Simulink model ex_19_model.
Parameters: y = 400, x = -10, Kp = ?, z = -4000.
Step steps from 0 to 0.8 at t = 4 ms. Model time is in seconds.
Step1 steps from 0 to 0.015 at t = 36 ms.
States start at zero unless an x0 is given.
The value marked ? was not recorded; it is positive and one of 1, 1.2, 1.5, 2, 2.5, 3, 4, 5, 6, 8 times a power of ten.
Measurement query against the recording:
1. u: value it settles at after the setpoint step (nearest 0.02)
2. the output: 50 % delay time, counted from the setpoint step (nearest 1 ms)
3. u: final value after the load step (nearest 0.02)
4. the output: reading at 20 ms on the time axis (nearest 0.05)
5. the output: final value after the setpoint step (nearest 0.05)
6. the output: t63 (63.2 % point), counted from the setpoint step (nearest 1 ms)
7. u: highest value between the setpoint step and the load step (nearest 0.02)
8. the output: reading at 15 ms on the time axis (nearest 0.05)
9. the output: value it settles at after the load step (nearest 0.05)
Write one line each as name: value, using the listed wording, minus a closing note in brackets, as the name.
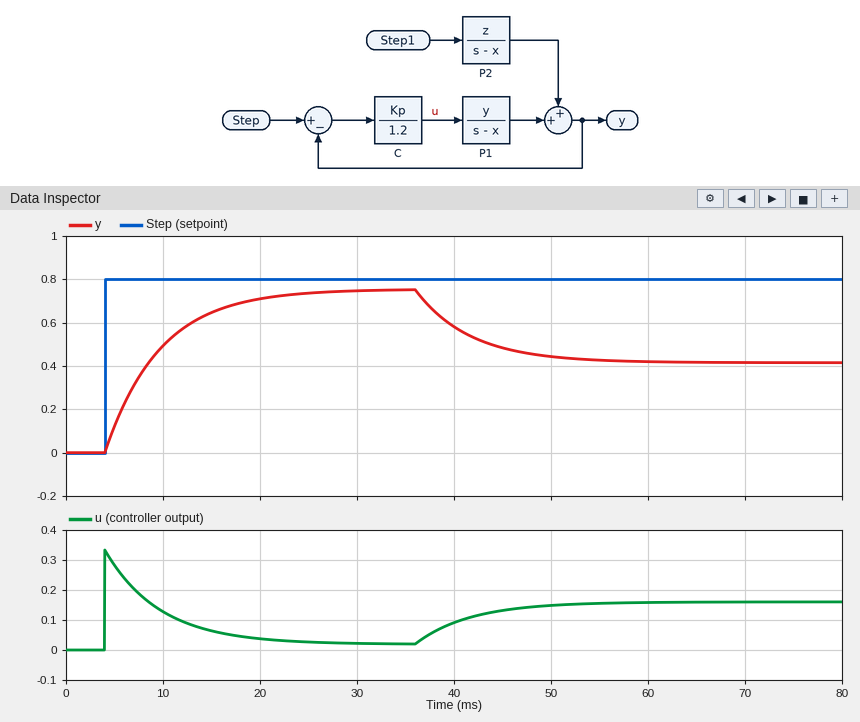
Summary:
u: value it settles at after the setpoint step: 0.02
the output: 50 % delay time, counted from the setpoint step: 4 ms
u: final value after the load step: 0.16
the output: reading at 20 ms on the time axis: 0.70
the output: final value after the setpoint step: 0.75
the output: t63 (63.2 % point), counted from the setpoint step: 6 ms
u: highest value between the setpoint step and the load step: 0.34
the output: reading at 15 ms on the time axis: 0.65
the output: value it settles at after the load step: 0.40
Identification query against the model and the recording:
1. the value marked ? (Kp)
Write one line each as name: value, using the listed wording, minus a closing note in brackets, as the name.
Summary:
the value marked ?: 0.5
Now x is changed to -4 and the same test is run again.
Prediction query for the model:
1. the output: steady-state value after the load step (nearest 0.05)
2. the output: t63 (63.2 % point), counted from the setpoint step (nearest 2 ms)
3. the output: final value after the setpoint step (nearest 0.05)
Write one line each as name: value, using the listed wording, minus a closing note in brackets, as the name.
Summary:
the output: steady-state value after the load step: 0.45
the output: t63 (63.2 % point), counted from the setpoint step: 6 ms
the output: final value after the setpoint step: 0.80
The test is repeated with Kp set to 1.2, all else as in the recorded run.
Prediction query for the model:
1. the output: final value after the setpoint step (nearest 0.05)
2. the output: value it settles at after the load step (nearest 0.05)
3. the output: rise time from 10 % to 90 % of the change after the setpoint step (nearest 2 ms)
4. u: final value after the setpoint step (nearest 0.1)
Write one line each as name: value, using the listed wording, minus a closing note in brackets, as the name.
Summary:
the output: final value after the setpoint step: 0.80
the output: value it settles at after the load step: 0.65
the output: rise time from 10 % to 90 % of the change after the setpoint step: 6 ms
u: final value after the setpoint step: 0.0
